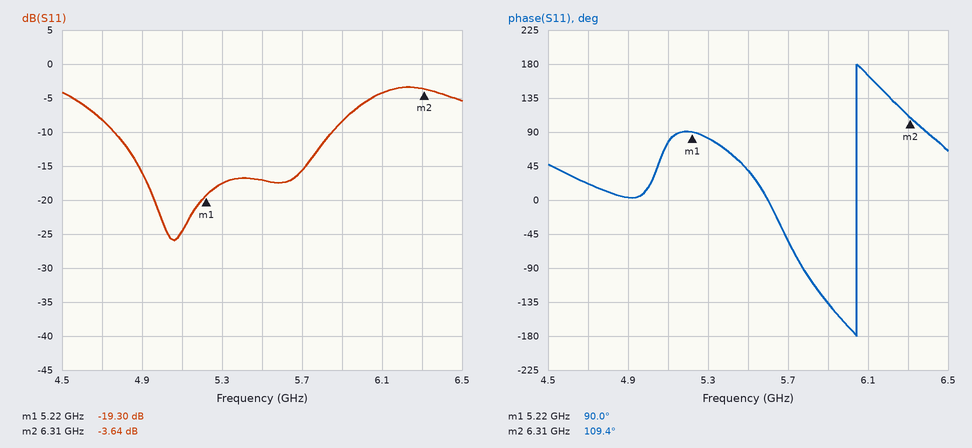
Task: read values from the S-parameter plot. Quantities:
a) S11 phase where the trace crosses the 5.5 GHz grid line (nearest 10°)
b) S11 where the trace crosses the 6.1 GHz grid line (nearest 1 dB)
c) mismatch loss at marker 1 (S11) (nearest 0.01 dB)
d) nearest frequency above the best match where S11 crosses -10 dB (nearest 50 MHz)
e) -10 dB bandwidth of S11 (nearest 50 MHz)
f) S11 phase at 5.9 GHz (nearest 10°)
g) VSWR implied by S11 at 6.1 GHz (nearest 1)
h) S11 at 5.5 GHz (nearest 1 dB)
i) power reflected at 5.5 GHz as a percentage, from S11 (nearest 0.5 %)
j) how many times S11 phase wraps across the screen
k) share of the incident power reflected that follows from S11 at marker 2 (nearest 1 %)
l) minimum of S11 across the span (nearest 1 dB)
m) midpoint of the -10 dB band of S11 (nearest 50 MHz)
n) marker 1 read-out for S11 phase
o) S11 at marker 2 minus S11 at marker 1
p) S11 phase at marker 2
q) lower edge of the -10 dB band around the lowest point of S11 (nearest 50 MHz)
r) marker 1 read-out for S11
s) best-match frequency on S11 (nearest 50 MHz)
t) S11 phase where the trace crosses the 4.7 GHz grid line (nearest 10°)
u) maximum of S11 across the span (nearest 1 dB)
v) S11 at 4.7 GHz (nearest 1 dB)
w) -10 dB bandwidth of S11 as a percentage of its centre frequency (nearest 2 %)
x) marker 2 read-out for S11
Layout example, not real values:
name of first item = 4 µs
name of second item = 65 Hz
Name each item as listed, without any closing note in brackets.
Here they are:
S11 phase where the trace crosses the 5.5 GHz grid line = 40°
S11 where the trace crosses the 6.1 GHz grid line = -4 dB
mismatch loss at marker 1 (S11) = 0.05 dB
nearest frequency above the best match where S11 crosses -10 dB = 5.85 GHz
-10 dB bandwidth of S11 = 1.10 GHz
S11 phase at 5.9 GHz = -140°
VSWR implied by S11 at 6.1 GHz = 4
S11 at 5.5 GHz = -17 dB
power reflected at 5.5 GHz as a percentage, from S11 = 2.0 %
how many times S11 phase wraps across the screen = 1
share of the incident power reflected that follows from S11 at marker 2 = 43 %
minimum of S11 across the span = -26 dB
midpoint of the -10 dB band of S11 = 5.30 GHz
marker 1 read-out for S11 phase = 90.0°
S11 at marker 2 minus S11 at marker 1 = 15.66 dB
S11 phase at marker 2 = 109.4°
lower edge of the -10 dB band around the lowest point of S11 = 4.75 GHz
marker 1 read-out for S11 = -19.30 dB
best-match frequency on S11 = 5.05 GHz
S11 phase where the trace crosses the 4.7 GHz grid line = 20°
maximum of S11 across the span = -3 dB
S11 at 4.7 GHz = -8 dB
-10 dB bandwidth of S11 as a percentage of its centre frequency = 20 %
marker 2 read-out for S11 = -3.64 dB
